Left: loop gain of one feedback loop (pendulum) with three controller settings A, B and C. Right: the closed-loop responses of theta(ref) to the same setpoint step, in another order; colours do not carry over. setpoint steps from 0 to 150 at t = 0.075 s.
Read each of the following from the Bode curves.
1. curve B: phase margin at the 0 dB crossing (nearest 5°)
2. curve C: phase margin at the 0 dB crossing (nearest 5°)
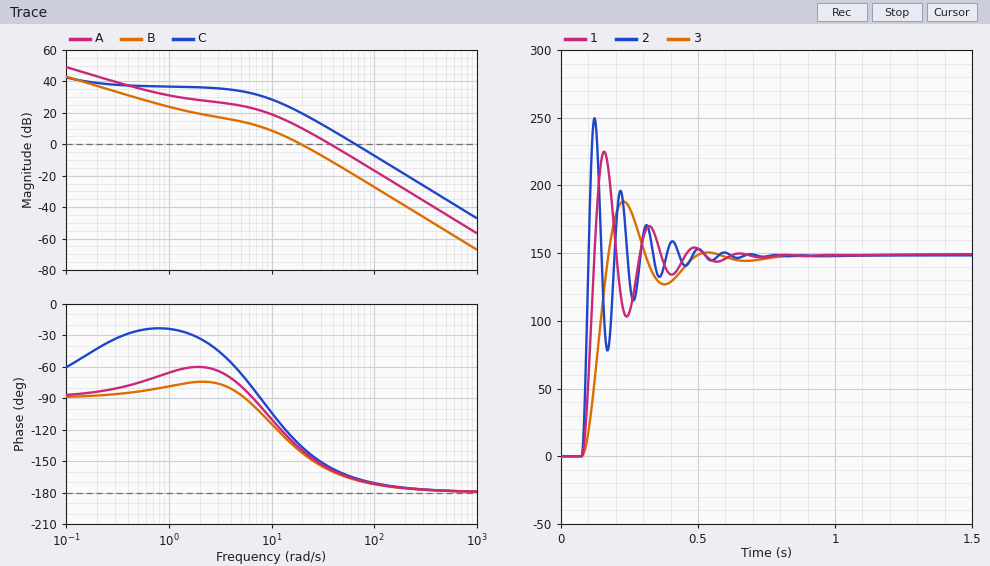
40°
15°
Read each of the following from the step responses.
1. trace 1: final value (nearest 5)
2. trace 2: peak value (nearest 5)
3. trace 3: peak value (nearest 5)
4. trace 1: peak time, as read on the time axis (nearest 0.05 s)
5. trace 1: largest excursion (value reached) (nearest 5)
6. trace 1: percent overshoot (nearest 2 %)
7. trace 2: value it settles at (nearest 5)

150
250
190
0.15 s
225
50 %
150
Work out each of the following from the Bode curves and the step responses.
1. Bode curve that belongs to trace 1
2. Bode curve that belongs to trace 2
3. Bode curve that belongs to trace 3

A
C
B
